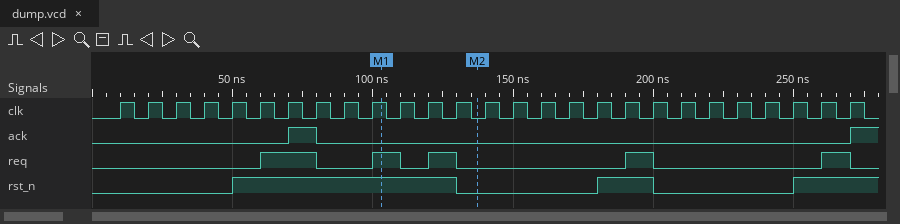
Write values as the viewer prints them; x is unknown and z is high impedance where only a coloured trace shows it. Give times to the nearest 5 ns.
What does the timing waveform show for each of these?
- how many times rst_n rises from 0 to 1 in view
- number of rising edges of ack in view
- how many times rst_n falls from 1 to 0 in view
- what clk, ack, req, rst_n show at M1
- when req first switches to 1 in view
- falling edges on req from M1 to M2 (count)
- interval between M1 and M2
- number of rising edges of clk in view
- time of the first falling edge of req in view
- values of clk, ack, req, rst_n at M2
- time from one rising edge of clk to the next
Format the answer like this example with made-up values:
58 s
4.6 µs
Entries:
3
2
2
clk=1, ack=0, req=1, rst_n=1
60 ns
2
35 ns
27
80 ns
clk=0, ack=0, req=0, rst_n=0
10 ns
